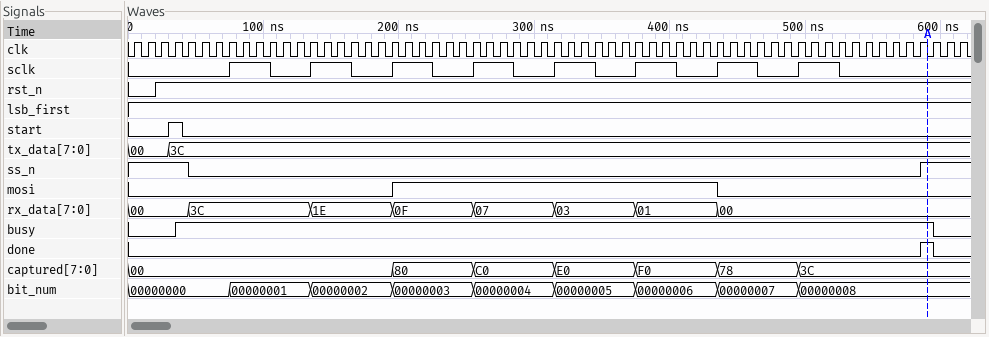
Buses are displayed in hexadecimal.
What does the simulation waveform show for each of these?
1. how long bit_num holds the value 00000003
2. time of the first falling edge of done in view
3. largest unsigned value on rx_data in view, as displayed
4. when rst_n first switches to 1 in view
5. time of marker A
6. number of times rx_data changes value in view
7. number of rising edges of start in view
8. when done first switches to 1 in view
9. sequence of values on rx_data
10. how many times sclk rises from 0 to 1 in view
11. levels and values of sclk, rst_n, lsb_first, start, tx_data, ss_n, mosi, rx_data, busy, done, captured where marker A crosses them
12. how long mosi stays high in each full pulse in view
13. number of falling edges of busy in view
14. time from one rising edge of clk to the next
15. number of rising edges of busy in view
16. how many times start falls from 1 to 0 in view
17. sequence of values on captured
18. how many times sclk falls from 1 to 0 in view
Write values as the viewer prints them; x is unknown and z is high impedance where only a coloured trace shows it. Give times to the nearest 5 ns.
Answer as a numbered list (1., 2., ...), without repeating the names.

1. 60 ns
2. 595 ns
3. 3C
4. 20 ns
5. 590 ns
6. 7
7. 1
8. 585 ns
9. 00, 3C, 1E, 0F, 07, 03, 01, 00
10. 8
11. sclk=0, rst_n=1, lsb_first=1, start=0, tx_data=3C, ss_n=1, mosi=0, rx_data=00, busy=1, done=1, captured=3C
12. 240 ns
13. 1
14. 10 ns
15. 1
16. 1
17. 00, 80, C0, E0, F0, 78, 3C
18. 8
